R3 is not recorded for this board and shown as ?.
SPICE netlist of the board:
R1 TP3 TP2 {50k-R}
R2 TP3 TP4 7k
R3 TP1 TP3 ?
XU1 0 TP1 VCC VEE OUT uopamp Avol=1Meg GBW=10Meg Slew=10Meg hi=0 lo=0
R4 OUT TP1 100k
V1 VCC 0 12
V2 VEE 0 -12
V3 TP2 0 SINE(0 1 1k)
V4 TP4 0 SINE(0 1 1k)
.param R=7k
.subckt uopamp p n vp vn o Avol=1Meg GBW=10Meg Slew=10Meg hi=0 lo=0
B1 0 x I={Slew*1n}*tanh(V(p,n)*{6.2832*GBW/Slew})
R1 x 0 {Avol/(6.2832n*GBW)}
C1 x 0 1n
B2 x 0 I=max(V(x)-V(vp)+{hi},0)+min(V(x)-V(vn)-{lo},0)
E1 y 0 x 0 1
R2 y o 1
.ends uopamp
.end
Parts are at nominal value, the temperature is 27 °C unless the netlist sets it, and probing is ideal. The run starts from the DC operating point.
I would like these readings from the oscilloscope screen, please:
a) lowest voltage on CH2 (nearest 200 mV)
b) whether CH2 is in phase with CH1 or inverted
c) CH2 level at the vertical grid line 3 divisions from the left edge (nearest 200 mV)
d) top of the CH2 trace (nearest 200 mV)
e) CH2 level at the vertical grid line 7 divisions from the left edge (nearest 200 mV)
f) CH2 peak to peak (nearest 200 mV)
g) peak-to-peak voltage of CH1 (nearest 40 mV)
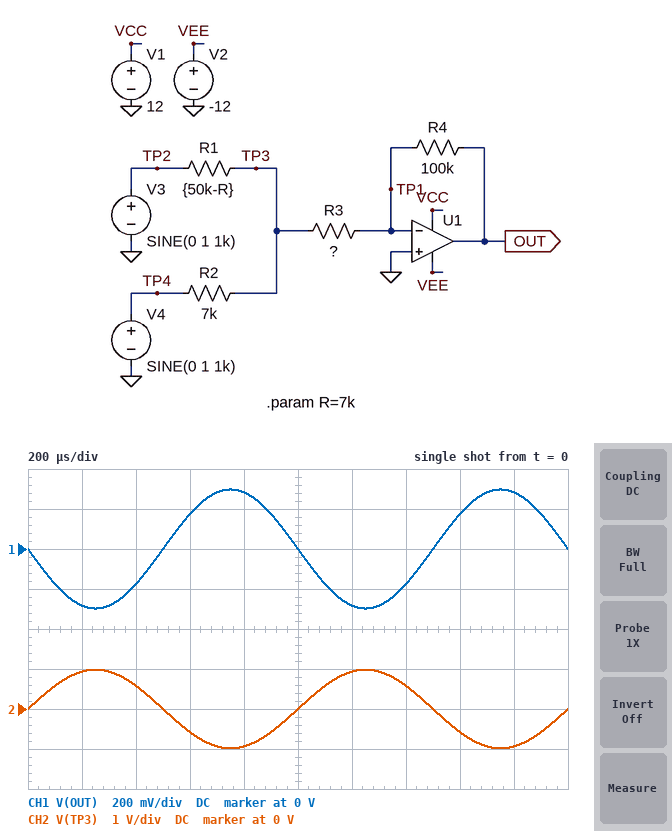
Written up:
-1.0 V
inverted
-600 mV
1.0 V
600 mV
2.0 V
600 mV
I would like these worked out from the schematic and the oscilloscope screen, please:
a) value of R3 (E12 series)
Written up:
330 kΩ
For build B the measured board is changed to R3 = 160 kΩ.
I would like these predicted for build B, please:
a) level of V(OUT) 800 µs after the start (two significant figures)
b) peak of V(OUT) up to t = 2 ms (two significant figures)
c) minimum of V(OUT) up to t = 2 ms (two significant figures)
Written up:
570 mV
600 mV
-600 mV
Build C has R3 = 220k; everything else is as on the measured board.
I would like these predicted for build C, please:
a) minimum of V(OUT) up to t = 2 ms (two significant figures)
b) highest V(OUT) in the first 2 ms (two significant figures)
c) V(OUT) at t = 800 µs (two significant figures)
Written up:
-440 mV
440 mV
420 mV
